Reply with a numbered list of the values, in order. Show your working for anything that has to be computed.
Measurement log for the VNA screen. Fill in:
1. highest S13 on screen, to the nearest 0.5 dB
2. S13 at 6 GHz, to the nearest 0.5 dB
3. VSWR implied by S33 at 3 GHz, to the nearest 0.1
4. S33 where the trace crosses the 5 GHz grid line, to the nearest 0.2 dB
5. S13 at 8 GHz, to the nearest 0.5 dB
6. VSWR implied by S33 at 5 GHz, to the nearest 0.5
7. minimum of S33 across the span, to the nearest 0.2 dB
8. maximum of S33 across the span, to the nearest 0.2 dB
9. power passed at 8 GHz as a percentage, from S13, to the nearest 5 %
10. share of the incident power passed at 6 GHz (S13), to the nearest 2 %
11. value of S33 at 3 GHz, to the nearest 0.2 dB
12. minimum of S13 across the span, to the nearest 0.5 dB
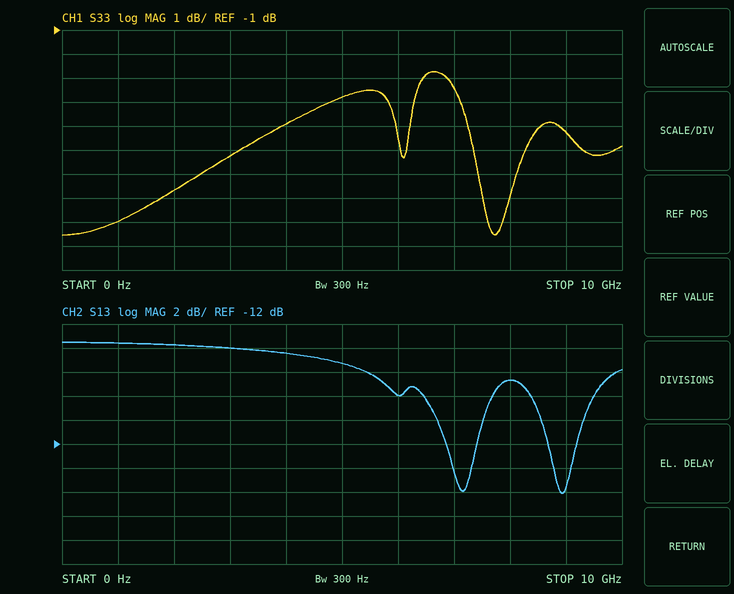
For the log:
1. -3.5 dB
2. -8.0 dB
3. |Γ| = 10^(-6.2/20) = 0.4898; VSWR = (1 + 0.4898)/(1 − 0.4898) ≈ 2.9
4. -3.8 dB
5. -6.5 dB
6. |Γ| = 10^(-3.8/20) = 0.6457; VSWR = (1 + 0.6457)/(1 − 0.6457) ≈ 4.64, so 4.5 to the nearest 0.5
7. -9.6 dB
8. -2.8 dB
9. 10^(-6.5/10) ≈ 22.4 %, so 20 % to the nearest 5 %
10. 10^(-8/10) ≈ 16 %
11. -6.2 dB
12. -16.0 dB
